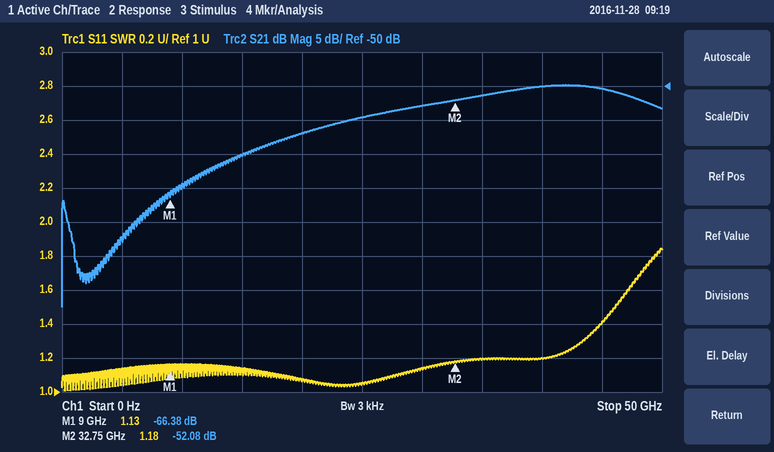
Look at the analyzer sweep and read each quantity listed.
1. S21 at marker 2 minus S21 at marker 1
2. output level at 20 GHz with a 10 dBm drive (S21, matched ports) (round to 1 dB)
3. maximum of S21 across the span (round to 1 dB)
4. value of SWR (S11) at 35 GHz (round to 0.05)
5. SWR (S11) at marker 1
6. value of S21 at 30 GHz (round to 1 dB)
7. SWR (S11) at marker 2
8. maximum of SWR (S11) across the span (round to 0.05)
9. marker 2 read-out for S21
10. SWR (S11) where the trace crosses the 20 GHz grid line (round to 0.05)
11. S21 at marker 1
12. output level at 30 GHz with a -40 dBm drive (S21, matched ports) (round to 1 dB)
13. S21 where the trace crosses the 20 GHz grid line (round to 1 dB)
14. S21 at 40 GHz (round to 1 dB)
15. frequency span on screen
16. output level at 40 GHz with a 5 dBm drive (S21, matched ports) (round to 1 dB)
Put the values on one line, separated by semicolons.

14.30 dB; -47 dBm; -50 dB; 1.20; 1.13; -53 dB; 1.18; 1.85; -52.08 dB; 1.05; -66.38 dB; -93 dBm; -57 dB; -50 dB; 50 GHz; -45 dBm
